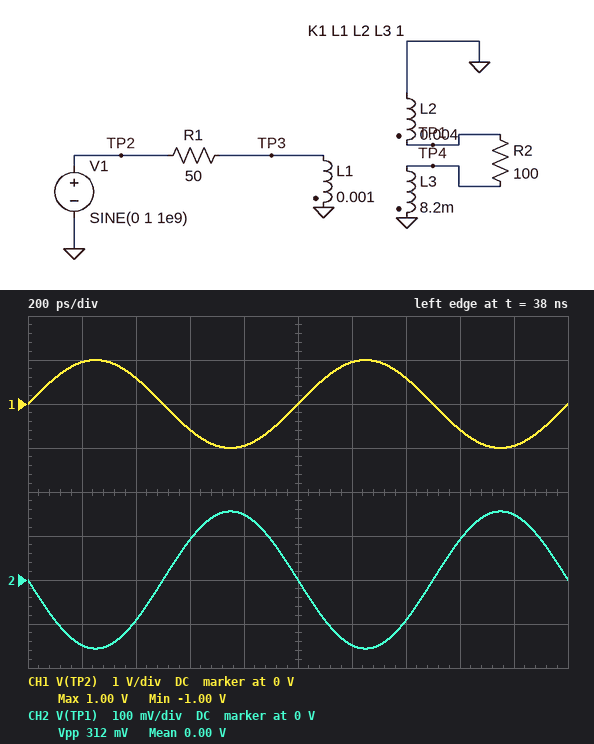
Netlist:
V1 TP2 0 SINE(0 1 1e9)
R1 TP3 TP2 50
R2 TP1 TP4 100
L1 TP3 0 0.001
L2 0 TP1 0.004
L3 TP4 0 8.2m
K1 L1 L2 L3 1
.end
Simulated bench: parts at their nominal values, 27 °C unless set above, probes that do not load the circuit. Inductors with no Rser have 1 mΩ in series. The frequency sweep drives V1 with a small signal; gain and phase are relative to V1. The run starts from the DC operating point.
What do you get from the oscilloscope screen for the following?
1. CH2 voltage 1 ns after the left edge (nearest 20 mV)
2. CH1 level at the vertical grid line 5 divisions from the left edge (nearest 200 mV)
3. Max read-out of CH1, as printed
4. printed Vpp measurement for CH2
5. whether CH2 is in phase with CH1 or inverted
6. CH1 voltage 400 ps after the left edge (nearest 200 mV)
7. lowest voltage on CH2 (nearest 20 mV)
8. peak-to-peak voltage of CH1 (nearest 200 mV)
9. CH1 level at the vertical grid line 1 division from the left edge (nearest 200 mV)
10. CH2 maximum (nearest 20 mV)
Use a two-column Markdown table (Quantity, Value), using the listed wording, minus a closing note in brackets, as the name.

| Quantity | Value |
|---|---|
| CH2 voltage 1 ns after the left edge | 0 V |
| CH1 level at the vertical grid line 5 divisions from the left edge | 0 V |
| Max read-out of CH1, as printed | 1.00 V |
| printed Vpp measurement for CH2 | 312 mV |
| whether CH2 is in phase with CH1 or inverted | inverted |
| CH1 voltage 400 ps after the left edge | 600 mV |
| lowest voltage on CH2 | -160 mV |
| peak-to-peak voltage of CH1 | 2.0 V |
| CH1 level at the vertical grid line 1 division from the left edge | 1.0 V |
| CH2 maximum | 160 mV |
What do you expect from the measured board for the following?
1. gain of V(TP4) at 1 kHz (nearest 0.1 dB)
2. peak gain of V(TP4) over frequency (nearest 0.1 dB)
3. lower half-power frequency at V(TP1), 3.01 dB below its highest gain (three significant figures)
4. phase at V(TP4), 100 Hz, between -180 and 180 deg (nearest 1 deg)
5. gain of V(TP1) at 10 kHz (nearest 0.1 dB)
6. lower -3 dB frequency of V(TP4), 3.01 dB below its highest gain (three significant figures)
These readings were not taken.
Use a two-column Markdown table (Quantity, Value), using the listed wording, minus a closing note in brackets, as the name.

| Quantity | Value |
|---|---|
| gain of V(TP4) at 1 kHz | -14.4 dB |
| peak gain of V(TP4) over frequency | -13.0 dB |
| lower half-power frequency at V(TP1), 3.01 dB below its highest gain | 620 Hz |
| phase at V(TP4), 100 Hz, between -180 and 180 deg | 81 deg |
| gain of V(TP1) at 10 kHz | -16.2 dB |
| lower -3 dB frequency of V(TP4), 3.01 dB below its highest gain | 620 Hz |
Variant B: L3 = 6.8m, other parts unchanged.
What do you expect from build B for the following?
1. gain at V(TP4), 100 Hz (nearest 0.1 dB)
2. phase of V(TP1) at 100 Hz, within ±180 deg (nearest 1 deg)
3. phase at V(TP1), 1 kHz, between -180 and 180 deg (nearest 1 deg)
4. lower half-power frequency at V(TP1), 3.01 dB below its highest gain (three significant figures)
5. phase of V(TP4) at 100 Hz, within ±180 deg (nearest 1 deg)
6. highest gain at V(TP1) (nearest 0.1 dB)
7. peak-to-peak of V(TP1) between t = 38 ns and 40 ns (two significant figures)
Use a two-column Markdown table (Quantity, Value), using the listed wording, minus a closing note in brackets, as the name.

| Quantity | Value |
|---|---|
| gain at V(TP4), 100 Hz | -29.8 dB |
| phase of V(TP1) at 100 Hz, within ±180 deg | -98 deg |
| phase at V(TP1), 1 kHz, between -180 and 180 deg | -146 deg |
| lower half-power frequency at V(TP1), 3.01 dB below its highest gain | 685 Hz |
| phase of V(TP4) at 100 Hz, within ±180 deg | 82 deg |
| highest gain at V(TP1) | -15.3 dB |
| peak-to-peak of V(TP1) between t = 38 ns and 40 ns | 340 mV |
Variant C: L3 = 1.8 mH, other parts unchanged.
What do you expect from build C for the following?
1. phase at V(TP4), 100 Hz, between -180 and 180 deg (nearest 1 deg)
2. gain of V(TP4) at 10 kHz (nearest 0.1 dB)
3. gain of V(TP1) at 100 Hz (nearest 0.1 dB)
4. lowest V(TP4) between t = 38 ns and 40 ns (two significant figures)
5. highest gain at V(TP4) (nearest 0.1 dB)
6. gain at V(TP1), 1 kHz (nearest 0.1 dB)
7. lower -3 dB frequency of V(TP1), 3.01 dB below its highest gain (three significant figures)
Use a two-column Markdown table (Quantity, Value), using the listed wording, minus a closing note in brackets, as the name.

| Quantity | Value |
|---|---|
| phase at V(TP4), 100 Hz, between -180 and 180 deg | 85 deg |
| gain of V(TP4) at 10 kHz | -13.9 dB |
| gain of V(TP1) at 100 Hz | -32.0 dB |
| lowest V(TP4) between t = 38 ns and 40 ns | -200 mV |
| highest gain at V(TP4) | -13.8 dB |
| gain at V(TP1), 1 kHz | -14.3 dB |
| lower -3 dB frequency of V(TP1), 3.01 dB below its highest gain | 1.21 kHz |
